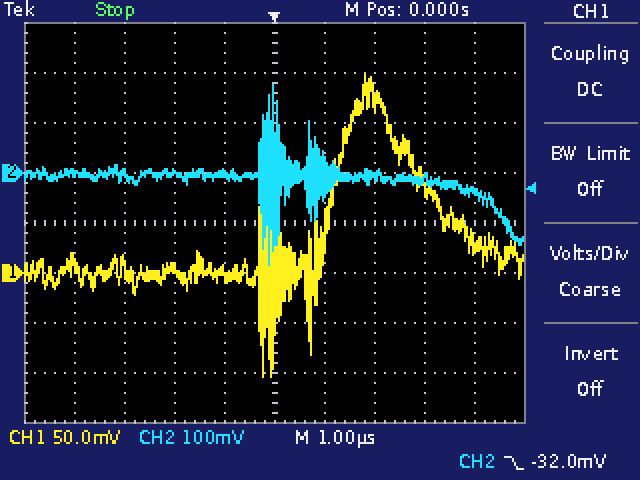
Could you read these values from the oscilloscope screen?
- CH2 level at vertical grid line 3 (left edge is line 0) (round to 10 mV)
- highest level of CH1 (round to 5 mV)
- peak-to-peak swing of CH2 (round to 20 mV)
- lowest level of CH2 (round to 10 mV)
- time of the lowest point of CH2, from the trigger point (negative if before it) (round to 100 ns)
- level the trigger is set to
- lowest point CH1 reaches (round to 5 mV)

0 mV
200 mV
360 mV
-180 mV
-100 ns
-32.0 mV
-105 mV
